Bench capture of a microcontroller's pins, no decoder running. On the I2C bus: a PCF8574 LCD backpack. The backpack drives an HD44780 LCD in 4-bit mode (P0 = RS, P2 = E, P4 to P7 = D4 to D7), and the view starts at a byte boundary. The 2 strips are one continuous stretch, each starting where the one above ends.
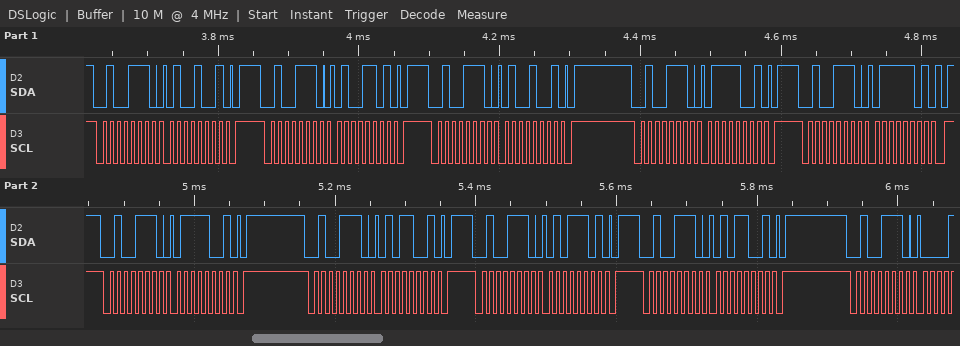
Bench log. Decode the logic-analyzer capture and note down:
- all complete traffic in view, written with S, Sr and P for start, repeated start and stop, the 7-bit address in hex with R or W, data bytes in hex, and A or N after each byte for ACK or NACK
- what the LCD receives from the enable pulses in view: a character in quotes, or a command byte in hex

S 27W A 49 A P S 27W A 4D A P S 27W A 49 A P S 27W A 79 A P S 27W A 7D A P S 27W A 79 A P S 27W A 59 A P S 27W A 5D A P S 27W A 59 A P S 27W A
'G'
